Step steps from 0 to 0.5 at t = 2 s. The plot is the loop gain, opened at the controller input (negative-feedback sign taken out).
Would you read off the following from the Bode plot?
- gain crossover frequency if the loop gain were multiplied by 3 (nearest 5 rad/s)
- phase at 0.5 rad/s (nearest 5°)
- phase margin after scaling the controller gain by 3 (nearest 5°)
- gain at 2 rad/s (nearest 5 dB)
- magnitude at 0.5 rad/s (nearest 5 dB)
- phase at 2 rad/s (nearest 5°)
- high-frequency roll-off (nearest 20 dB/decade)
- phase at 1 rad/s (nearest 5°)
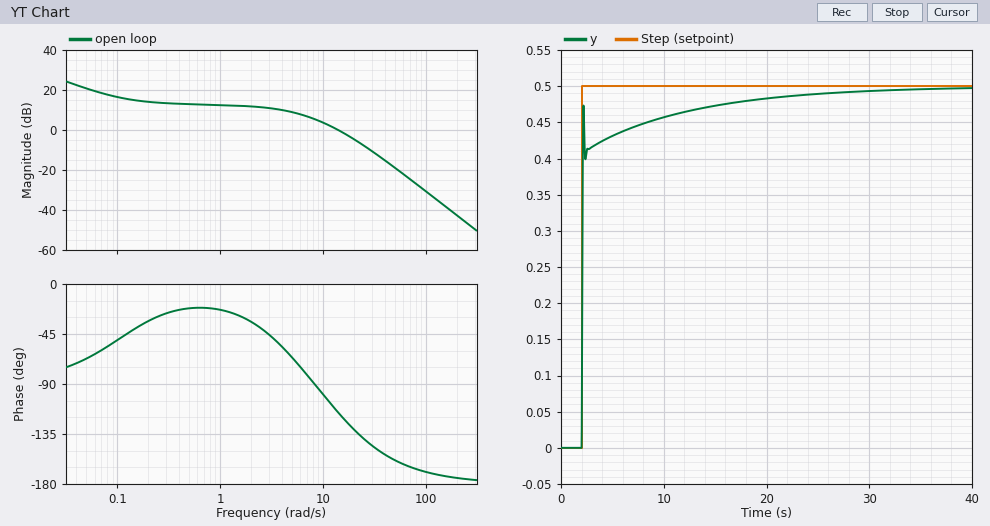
30 rad/s
-20°
35°
10 dB
15 dB
-35°
-40 dB/decade
-25°
